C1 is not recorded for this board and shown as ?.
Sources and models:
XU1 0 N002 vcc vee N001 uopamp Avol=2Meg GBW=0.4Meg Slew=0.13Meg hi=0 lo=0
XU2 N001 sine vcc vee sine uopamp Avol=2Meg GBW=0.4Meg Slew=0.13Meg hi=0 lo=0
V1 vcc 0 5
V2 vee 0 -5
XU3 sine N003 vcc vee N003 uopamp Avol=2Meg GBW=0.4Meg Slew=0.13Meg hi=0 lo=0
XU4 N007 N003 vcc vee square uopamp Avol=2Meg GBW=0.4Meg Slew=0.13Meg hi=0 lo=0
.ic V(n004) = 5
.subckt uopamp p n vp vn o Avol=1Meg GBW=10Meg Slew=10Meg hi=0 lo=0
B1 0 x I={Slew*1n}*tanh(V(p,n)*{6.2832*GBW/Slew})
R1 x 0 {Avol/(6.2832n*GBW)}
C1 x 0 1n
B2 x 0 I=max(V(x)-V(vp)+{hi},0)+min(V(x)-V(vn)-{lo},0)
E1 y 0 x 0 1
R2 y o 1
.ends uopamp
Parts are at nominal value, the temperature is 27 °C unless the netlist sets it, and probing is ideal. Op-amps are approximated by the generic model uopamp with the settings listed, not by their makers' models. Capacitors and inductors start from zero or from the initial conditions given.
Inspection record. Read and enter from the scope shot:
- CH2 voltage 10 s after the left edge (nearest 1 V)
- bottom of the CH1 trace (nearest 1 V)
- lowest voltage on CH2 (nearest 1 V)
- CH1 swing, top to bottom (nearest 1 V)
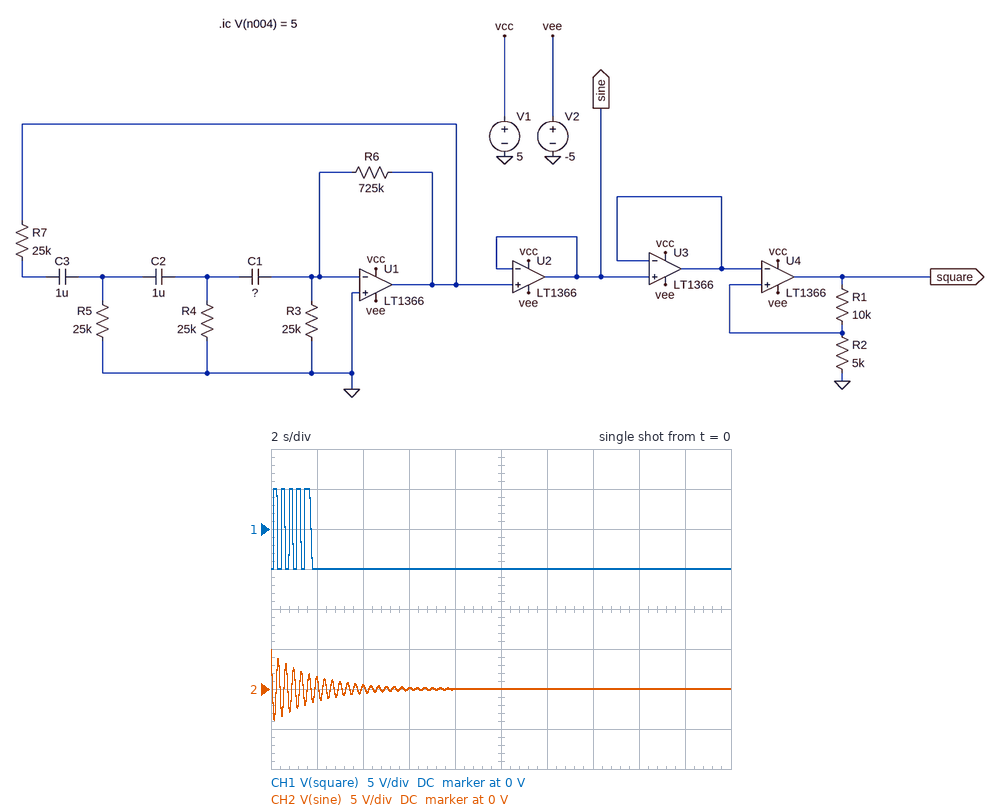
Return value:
0 V
-5 V
-4 V
10 V
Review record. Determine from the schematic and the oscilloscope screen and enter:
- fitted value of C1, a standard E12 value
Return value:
680 nF
